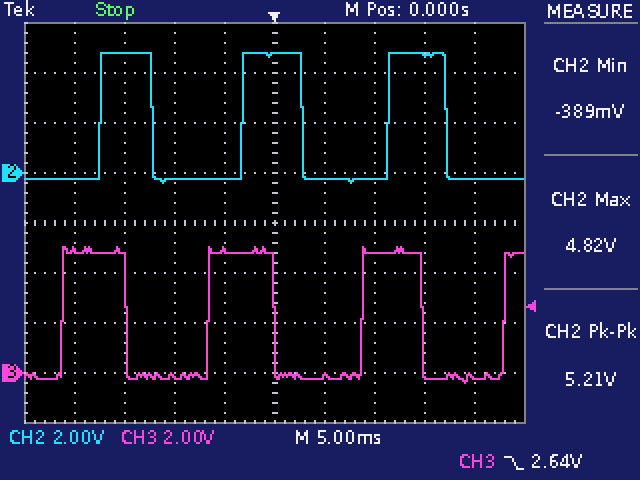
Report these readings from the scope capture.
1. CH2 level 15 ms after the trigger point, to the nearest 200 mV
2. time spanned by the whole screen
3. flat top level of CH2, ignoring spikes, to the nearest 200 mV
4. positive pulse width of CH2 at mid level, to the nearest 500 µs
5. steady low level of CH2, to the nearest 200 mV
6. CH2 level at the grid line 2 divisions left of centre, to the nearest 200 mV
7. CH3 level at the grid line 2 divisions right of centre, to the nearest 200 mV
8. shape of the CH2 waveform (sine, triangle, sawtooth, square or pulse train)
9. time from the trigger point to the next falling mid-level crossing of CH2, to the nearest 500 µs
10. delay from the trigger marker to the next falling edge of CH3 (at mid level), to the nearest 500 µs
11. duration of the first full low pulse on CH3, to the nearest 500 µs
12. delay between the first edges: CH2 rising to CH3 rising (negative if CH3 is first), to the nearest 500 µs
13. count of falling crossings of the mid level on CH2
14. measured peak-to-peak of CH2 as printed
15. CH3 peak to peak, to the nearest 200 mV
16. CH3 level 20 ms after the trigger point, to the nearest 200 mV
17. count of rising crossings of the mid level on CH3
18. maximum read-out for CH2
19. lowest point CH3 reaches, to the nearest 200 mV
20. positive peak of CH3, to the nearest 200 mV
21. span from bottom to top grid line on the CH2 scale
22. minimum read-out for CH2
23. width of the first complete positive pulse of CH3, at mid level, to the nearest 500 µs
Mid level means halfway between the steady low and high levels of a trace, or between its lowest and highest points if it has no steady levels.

4.8 V
50 ms
4.8 V
5.5 ms
-200 mV
-200 mV
4.8 V
pulse train
3.0 ms
15.0 ms
8.0 ms
-4.0 ms
3
5.21 V
5.4 V
-200 mV
4
4.82 V
-400 mV
5.0 V
16 V
-389 mV
6.5 ms
